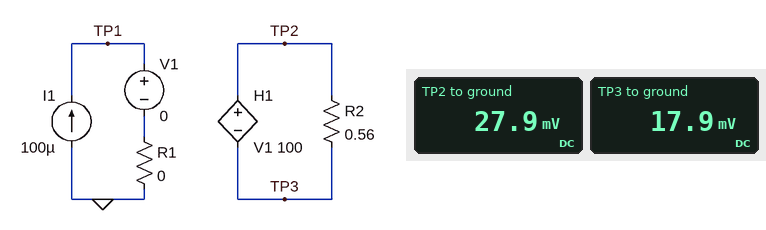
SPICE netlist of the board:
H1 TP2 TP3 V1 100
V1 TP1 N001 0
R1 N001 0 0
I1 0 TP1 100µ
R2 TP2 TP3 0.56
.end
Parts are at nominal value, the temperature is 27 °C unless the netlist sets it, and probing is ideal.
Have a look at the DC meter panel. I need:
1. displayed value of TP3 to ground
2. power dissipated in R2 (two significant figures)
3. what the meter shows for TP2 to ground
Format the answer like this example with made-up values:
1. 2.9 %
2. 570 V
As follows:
1. 17.9 mV
2. 180 µW
3. 27.9 mV
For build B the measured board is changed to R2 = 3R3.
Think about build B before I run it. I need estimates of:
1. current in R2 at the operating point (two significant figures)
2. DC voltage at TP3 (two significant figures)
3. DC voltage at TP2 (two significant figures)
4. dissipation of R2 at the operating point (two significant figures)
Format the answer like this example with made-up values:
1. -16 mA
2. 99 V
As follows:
1. 3.0 mA
2. 3.0 mV
3. 13 mV
4. 30 µW
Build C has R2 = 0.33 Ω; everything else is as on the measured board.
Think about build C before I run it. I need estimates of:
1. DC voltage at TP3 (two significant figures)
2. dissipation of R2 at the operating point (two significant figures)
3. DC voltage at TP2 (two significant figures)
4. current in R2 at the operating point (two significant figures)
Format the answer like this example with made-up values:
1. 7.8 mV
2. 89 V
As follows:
1. 30 mV
2. 300 µW
3. 40 mV
4. 30 mA
